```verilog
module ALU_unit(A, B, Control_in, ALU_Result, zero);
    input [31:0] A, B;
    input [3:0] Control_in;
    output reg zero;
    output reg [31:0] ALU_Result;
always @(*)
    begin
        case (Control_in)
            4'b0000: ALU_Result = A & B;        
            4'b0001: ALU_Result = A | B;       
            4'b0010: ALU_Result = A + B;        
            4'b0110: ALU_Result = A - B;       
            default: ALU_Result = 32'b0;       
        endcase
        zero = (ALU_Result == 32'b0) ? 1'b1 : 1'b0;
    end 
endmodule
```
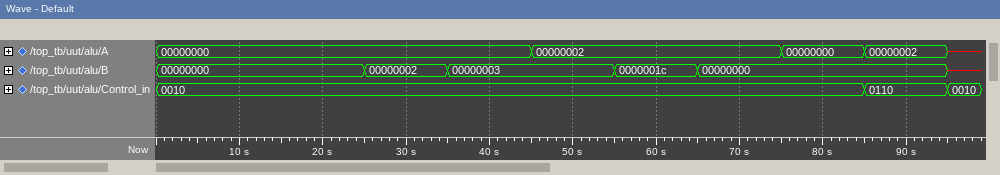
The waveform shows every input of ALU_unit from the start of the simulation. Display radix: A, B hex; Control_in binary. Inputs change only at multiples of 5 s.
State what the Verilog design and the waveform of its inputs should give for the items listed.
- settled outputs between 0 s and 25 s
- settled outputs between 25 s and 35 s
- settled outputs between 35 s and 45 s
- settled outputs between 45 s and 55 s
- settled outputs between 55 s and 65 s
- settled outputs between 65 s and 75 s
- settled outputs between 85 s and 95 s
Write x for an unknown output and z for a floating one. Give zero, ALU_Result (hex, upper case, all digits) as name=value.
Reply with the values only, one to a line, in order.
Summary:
zero=1, ALU_Result=00000000
zero=0, ALU_Result=00000002
zero=0, ALU_Result=00000003
zero=0, ALU_Result=00000005
zero=0, ALU_Result=0000001E
zero=0, ALU_Result=00000002
zero=0, ALU_Result=00000002
